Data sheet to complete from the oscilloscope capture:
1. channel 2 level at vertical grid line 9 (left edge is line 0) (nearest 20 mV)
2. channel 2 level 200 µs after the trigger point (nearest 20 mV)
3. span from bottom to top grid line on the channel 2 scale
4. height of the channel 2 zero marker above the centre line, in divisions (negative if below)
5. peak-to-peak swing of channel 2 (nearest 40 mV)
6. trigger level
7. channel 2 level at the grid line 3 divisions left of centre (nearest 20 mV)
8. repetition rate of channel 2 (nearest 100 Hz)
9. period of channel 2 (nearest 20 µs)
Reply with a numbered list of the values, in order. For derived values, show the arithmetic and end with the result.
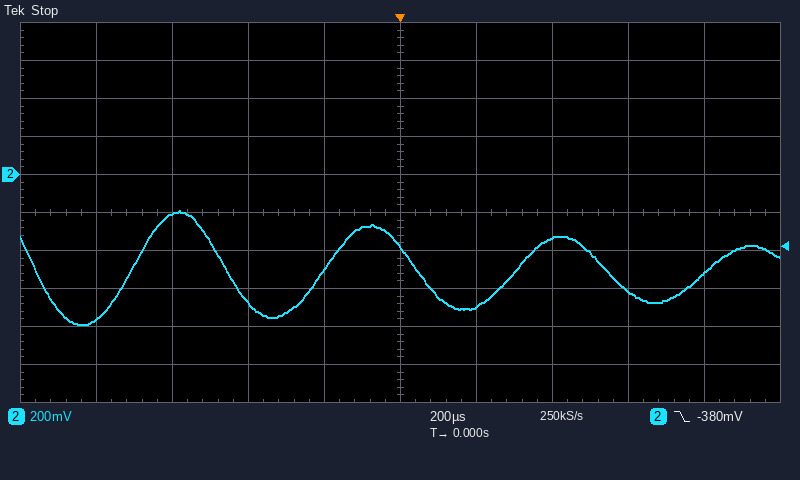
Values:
1. -520 mV
2. -700 mV
3. 2 V
4. +1.0 div
5. 600 mV
6. -380 mV
7. -200 mV
8. 1 / 500 µs ≈ 2.0 kHz
9. 500 µs
